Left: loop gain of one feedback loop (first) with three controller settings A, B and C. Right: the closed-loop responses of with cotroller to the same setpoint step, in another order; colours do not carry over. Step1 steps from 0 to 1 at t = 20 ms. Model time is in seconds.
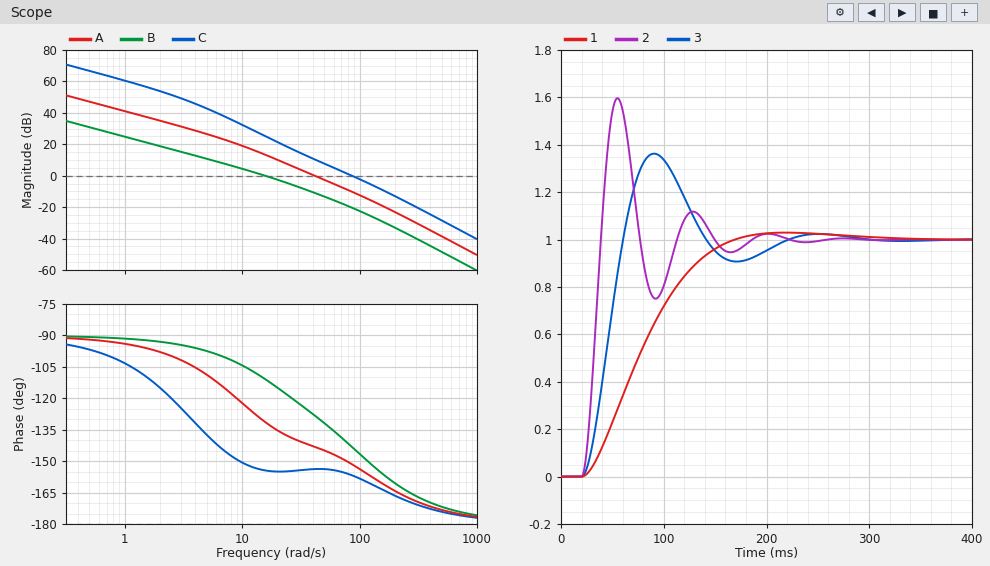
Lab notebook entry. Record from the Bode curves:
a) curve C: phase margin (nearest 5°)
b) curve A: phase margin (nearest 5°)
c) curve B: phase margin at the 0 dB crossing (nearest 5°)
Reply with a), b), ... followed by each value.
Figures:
a) 25°
b) 35°
c) 70°
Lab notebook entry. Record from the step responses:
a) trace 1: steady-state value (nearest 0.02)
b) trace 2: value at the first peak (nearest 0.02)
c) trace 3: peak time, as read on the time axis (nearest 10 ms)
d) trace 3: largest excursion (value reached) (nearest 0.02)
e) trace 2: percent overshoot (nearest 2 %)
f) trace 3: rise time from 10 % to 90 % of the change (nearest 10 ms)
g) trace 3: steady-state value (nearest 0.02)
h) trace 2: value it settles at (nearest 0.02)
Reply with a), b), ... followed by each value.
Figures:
a) 1.00
b) 1.60
c) 90 ms
d) 1.36
e) 60 %
f) 30 ms
g) 1.00
h) 1.00
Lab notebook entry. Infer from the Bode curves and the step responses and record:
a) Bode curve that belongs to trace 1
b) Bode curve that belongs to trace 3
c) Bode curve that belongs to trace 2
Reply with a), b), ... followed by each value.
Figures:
a) B
b) A
c) C
